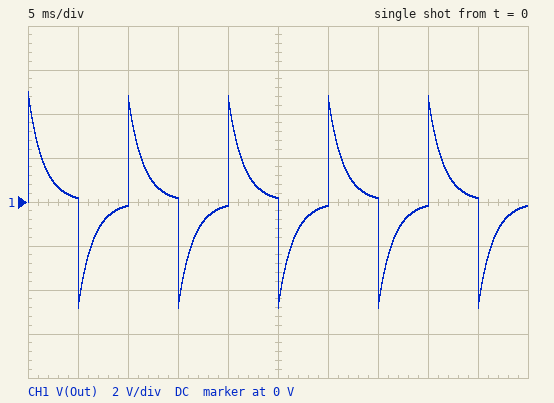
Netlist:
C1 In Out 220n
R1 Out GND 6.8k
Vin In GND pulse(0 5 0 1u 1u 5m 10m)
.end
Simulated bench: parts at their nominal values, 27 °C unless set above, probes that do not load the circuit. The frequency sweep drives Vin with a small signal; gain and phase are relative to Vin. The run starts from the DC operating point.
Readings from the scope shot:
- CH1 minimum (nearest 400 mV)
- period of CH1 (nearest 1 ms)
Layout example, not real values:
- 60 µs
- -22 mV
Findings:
- -4.8 V
- 10 ms
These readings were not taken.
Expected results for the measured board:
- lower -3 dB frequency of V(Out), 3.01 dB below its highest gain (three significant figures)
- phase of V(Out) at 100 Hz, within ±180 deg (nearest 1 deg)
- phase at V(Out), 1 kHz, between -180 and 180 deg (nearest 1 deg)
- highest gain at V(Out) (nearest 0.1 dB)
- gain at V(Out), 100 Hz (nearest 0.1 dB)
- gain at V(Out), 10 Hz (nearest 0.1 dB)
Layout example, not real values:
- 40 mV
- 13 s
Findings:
- 106 Hz
- 47 deg
- 6 deg
- 0 dB
- -3.3 dB
- -20.6 dB
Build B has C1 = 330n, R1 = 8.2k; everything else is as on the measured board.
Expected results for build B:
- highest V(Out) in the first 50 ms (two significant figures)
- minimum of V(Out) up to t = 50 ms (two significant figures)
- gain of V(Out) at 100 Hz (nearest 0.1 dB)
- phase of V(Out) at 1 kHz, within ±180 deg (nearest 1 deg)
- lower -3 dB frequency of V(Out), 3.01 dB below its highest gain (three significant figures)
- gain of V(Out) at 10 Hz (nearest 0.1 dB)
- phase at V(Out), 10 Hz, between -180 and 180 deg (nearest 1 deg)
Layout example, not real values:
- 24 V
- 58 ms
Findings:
- 5.0 V
- -4.3 V
- -1.3 dB
- 3 deg
- 58.8 Hz
- -15.5 dB
- 80 deg
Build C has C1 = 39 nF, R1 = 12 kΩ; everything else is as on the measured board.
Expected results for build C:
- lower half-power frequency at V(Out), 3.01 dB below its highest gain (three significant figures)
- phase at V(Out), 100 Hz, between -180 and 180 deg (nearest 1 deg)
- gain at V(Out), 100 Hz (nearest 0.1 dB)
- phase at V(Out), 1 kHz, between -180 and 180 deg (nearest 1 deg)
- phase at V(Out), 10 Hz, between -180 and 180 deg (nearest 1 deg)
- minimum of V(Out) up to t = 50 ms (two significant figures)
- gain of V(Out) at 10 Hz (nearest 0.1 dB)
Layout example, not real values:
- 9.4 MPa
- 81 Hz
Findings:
- 340 Hz
- 74 deg
- -11.0 dB
- 19 deg
- 88 deg
- -5.0 V
- -30.6 dB
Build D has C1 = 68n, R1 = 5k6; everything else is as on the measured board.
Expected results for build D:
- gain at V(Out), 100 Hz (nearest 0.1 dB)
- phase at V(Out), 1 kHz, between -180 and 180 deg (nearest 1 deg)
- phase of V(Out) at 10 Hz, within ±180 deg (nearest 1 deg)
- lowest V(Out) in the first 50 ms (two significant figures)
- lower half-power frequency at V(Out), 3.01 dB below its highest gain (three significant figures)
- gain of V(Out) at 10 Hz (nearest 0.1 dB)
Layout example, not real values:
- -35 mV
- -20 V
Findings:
- -12.7 dB
- 23 deg
- 89 deg
- -5.0 V
- 418 Hz
- -32.4 dB
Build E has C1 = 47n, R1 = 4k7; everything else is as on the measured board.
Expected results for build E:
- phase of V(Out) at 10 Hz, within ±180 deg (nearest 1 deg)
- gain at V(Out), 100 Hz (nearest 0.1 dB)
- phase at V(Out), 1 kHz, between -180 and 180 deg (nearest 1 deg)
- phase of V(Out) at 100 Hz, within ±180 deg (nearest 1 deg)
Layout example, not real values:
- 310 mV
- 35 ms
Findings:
- 89 deg
- -17.2 dB
- 36 deg
- 82 deg
